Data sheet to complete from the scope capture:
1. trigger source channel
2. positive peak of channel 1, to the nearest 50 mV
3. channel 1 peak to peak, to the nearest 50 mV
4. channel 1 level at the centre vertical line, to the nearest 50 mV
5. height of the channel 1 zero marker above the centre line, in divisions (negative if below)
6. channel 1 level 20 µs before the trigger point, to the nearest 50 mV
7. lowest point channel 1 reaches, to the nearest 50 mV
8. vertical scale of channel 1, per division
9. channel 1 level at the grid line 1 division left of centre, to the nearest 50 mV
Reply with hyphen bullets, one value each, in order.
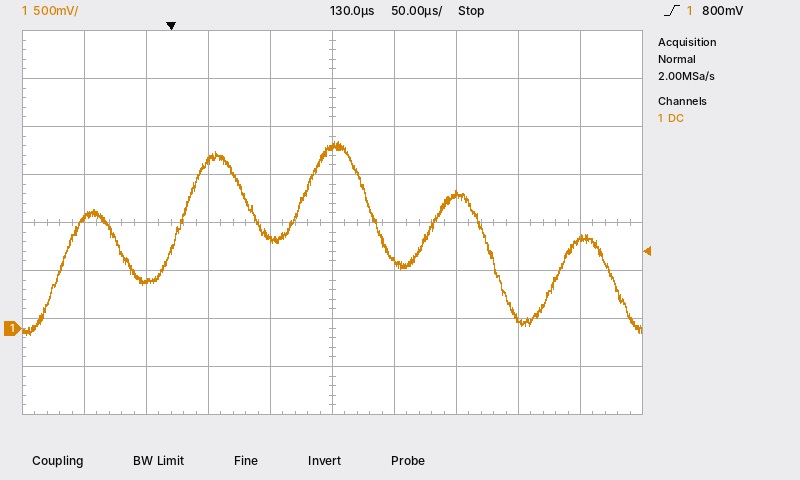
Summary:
- channel 1
- 1.95 V
- 2.00 V
- 1.90 V
- -2.2 div
- 500 mV
- -50 mV
- 500 mV
- 950 mV
